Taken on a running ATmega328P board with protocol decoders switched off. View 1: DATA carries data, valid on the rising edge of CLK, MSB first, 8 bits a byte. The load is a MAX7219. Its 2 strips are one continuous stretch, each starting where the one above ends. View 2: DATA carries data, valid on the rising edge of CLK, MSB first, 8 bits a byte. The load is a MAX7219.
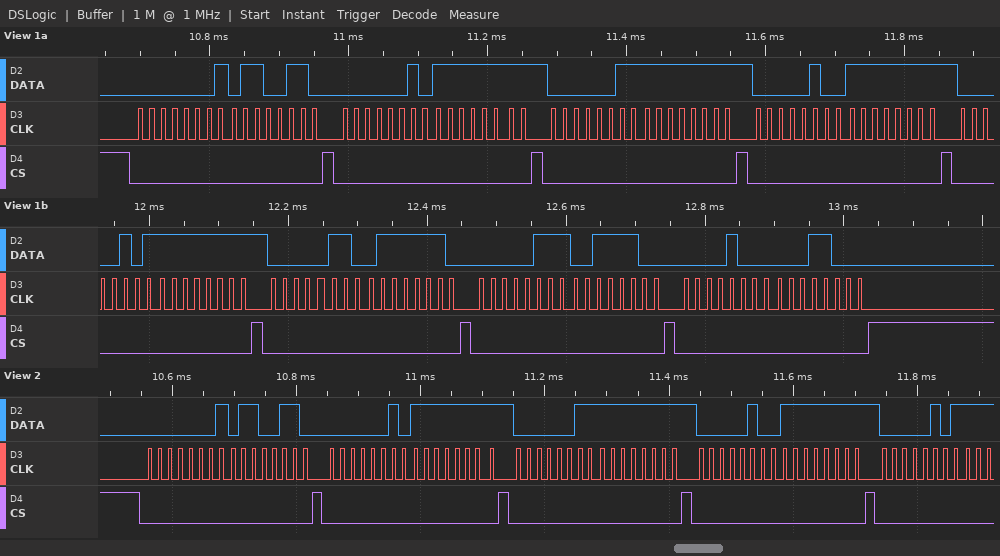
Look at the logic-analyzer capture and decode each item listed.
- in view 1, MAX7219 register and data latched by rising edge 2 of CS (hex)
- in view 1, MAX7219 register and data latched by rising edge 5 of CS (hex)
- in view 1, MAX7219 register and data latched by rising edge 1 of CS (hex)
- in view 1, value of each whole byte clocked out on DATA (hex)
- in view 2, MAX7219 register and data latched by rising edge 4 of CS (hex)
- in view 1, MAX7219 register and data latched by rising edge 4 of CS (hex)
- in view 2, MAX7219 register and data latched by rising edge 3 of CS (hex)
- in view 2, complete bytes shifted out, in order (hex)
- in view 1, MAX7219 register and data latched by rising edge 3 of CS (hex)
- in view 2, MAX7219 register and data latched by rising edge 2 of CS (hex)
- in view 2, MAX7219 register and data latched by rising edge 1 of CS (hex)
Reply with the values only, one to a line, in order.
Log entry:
register 0x2, data 0xFF
register 0x5, data 0xFF
register 0x1, data 0x66
01 66 02 FF 03 FF 04 FF 05 FF 06 7E 07 3C 08 18
register 0x4, data 0xFF
register 0x4, data 0xFF
register 0x3, data 0xFF
0x01 0x66 0x02 0xFF 0x03 0xFF 0x04 0xFF 0x05
register 0x3, data 0xFF
register 0x2, data 0xFF
register 0x1, data 0x66
